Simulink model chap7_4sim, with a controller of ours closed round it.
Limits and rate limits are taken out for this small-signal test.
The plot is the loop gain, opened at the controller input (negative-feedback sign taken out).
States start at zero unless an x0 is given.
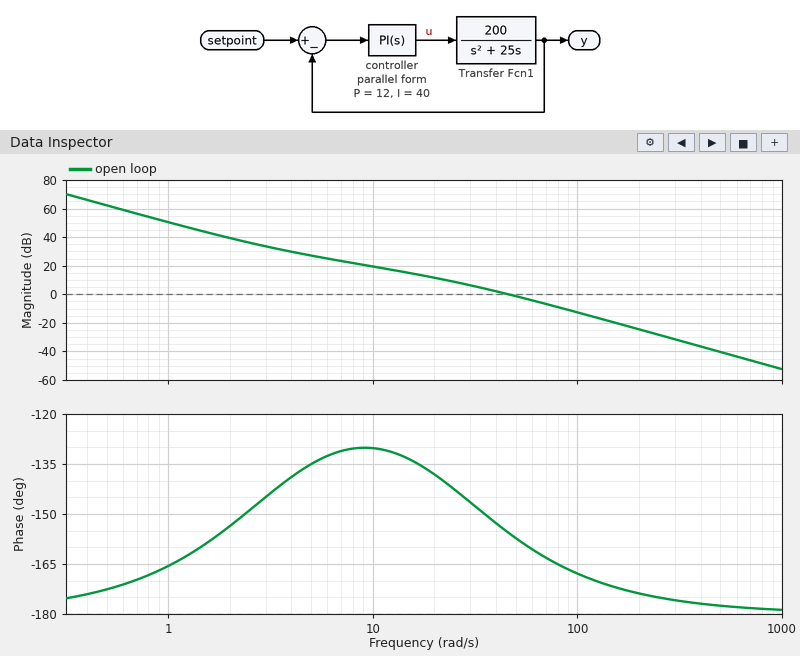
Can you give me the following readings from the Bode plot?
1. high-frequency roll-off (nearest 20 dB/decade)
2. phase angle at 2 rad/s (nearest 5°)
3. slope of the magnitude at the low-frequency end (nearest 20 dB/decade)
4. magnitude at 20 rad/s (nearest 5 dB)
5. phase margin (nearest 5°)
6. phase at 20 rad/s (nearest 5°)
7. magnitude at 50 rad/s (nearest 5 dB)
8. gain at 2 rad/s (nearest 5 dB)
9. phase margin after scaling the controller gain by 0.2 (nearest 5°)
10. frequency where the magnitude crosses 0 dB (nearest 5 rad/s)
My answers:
-40 dB/decade
-155°
-40 dB/decade
10 dB
25°
-140°
0 dB
40 dB
45°
45 rad/s
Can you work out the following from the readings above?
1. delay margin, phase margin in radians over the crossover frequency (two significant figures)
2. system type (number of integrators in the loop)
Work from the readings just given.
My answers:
0.0097 s
2
